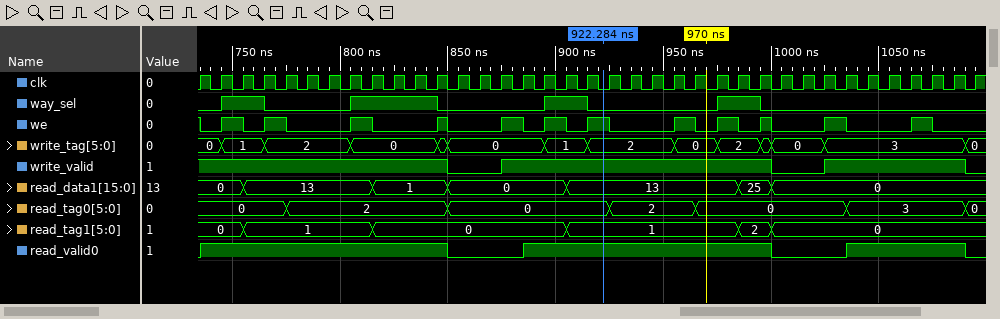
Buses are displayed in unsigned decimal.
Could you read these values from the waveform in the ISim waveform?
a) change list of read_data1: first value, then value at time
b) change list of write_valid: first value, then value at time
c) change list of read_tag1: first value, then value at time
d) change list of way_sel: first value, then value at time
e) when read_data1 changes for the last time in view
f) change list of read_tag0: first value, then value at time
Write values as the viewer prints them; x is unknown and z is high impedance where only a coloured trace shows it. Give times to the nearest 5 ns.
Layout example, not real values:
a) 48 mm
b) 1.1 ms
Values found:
a) 0, 13 at 755 ns, 1 at 815 ns, 0 at 850 ns, 13 at 905 ns, 25 at 985 ns, 0 at 1000 ns
b) 1, 0 at 850 ns, 1 at 875 ns, 0 at 1000 ns, 1 at 1025 ns, 0 at 1090 ns
c) 0, 1 at 755 ns, 0 at 815 ns, 1 at 905 ns, 2 at 985 ns, 0 at 1000 ns
d) 0, 1 at 745 ns, 0 at 765 ns, 1 at 805 ns, 0 at 845 ns, 1 at 895 ns, 0 at 915 ns, 1 at 975 ns, 0 at 995 ns
e) 1000 ns
f) 0, 2 at 775 ns, 0 at 850 ns, 2 at 925 ns, 0 at 965 ns, 3 at 1035 ns, 0 at 1090 ns
